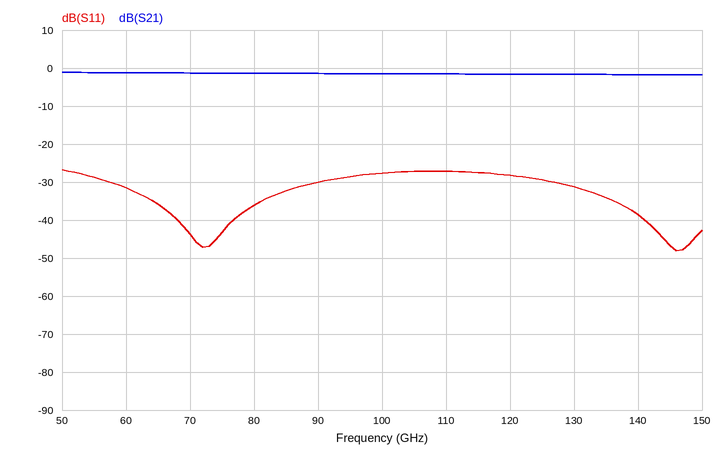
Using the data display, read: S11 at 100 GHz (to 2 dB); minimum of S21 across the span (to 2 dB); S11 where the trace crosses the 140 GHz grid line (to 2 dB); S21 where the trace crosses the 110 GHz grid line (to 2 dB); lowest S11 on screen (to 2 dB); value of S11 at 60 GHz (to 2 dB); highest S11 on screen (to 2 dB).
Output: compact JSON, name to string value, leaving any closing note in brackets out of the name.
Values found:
{"S11 at 100 GHz": "-28 dB", "minimum of S21 across the span": "-2 dB", "S11 where the trace crosses the 140 GHz grid line": "-38 dB", "S21 where the trace crosses the 110 GHz grid line": "-2 dB", "lowest S11 on screen": "-48 dB", "value of S11 at 60 GHz": "-32 dB", "highest S11 on screen": "-26 dB"}
